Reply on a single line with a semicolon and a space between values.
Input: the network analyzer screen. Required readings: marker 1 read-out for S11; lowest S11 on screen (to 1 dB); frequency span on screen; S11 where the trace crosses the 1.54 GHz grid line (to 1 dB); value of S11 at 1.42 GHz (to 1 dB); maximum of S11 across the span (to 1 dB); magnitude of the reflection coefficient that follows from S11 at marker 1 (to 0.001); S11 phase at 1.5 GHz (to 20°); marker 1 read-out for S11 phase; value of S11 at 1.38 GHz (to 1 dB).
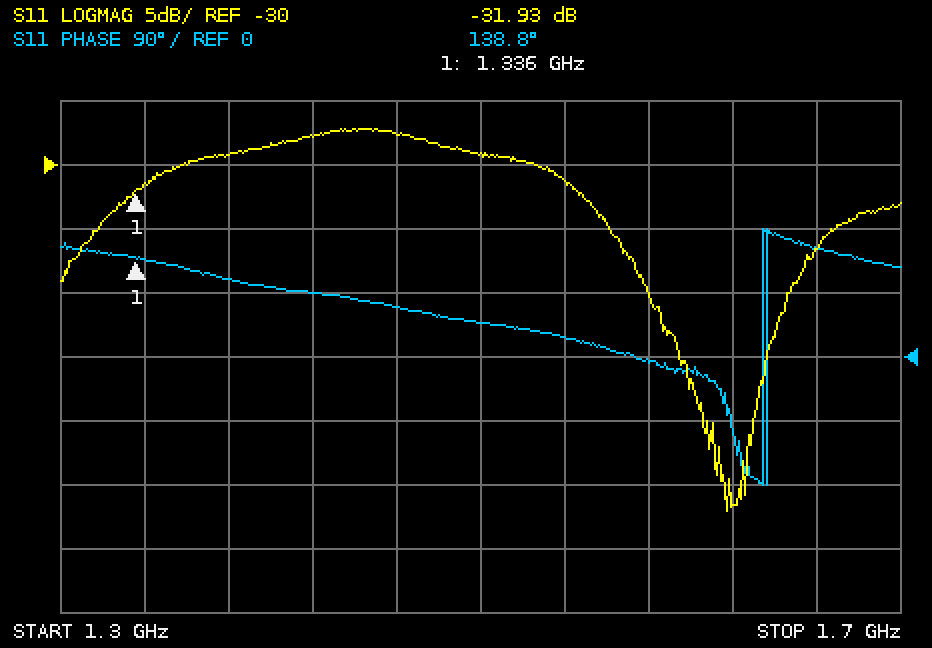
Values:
-31.93 dB; -57 dB; 400 MHz; -31 dB; -28 dB; -27 dB; 0.025; 40°; 138.8°; -29 dB
